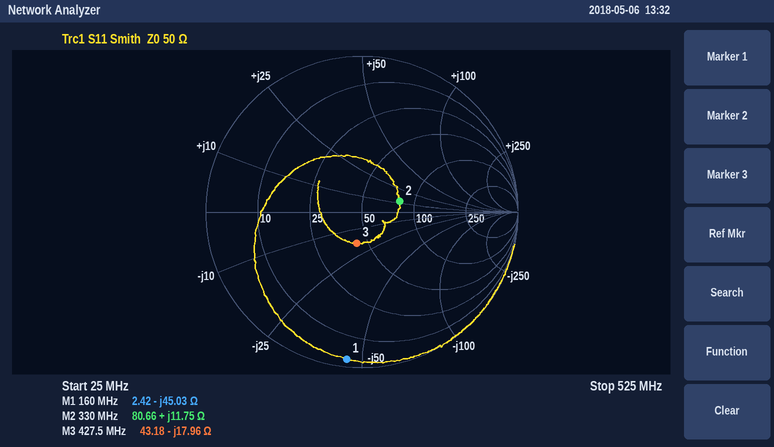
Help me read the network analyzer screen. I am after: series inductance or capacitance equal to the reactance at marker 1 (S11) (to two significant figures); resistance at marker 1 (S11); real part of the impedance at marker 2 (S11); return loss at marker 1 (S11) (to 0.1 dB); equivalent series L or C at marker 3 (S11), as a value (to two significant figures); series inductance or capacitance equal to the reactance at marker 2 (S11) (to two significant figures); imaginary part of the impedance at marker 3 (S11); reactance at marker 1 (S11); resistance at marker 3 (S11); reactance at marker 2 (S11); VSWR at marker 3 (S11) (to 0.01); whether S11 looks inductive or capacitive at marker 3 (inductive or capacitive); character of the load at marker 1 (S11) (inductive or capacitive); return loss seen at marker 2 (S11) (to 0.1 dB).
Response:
22 pF
2.42 Ω
80.66 Ω
0.5 dB
21 pF
5.7 nH
-17.96 Ω
-45.03 Ω
43.18 Ω
+11.75 Ω
1.51
capacitive
capacitive
12.0 dB
